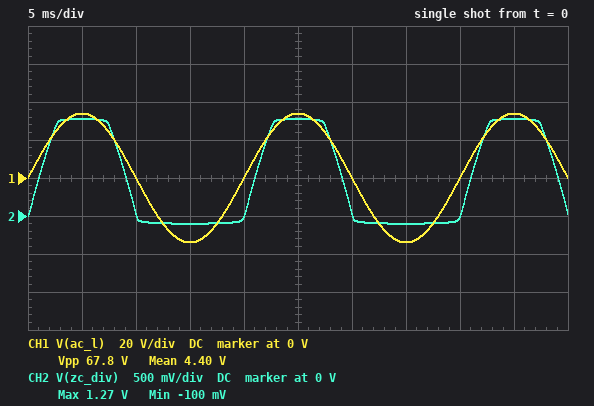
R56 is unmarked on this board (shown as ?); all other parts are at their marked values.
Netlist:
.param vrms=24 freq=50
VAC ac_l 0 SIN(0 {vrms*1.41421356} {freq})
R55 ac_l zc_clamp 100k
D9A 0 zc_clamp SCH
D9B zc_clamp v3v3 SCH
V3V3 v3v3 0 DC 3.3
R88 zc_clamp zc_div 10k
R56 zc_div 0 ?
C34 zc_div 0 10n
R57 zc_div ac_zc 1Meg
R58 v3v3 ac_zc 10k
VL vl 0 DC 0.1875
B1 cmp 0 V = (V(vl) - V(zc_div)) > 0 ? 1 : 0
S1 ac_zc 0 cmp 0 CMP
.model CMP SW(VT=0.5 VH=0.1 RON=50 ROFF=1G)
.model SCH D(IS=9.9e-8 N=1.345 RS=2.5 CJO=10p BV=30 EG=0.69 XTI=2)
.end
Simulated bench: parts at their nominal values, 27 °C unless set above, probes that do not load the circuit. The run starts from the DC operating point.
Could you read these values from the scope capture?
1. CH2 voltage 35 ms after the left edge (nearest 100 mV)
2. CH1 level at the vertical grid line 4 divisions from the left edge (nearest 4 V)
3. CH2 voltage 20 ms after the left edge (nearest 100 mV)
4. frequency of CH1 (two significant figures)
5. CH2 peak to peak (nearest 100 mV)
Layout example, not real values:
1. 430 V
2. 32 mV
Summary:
1. -100 mV
2. 0 V
3. 0 V
4. 50 Hz
5. 1.4 V
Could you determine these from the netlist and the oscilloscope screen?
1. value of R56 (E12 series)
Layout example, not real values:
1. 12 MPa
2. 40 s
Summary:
1. 5.6 kΩ
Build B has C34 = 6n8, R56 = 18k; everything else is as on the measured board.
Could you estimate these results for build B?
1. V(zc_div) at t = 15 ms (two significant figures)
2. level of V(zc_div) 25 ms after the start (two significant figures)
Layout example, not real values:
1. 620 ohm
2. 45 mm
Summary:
1. -180 mV
2. 2.3 V
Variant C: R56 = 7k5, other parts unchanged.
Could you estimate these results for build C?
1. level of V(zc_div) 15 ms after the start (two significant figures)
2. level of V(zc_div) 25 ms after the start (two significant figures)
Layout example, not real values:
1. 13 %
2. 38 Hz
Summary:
1. -120 mV
2. 1.5 V
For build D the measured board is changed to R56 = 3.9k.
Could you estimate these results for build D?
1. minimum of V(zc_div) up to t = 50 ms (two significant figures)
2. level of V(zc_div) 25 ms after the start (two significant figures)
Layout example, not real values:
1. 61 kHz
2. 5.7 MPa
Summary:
1. -79 mV
2. 990 mV
